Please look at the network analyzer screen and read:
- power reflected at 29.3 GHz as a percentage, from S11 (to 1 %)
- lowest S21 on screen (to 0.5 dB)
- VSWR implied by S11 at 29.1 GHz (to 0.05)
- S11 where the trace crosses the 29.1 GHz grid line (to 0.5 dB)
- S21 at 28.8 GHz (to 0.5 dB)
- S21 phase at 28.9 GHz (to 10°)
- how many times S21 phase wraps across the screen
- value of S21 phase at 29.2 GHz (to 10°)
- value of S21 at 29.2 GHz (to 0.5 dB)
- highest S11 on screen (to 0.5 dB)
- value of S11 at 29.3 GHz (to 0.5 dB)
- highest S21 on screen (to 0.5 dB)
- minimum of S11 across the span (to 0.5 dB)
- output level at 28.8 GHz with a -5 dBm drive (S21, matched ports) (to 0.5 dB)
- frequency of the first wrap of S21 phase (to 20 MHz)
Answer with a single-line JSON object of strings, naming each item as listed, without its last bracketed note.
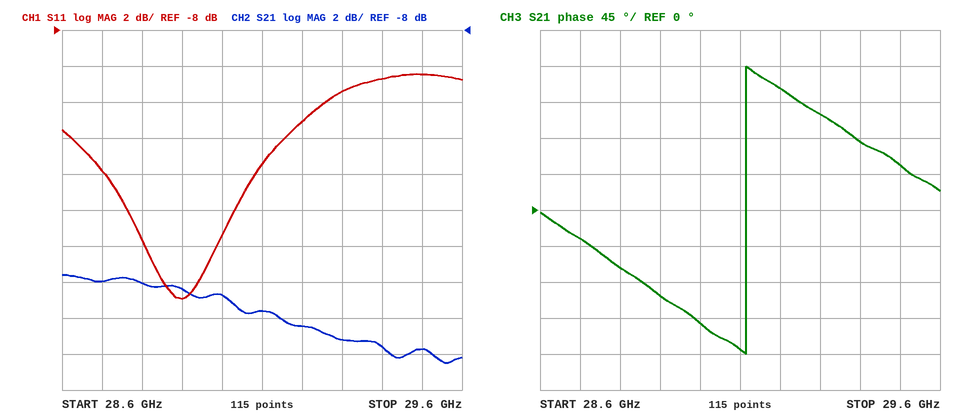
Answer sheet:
{"power reflected at 29.3 GHz as a percentage, from S11": "7 %", "lowest S21 on screen": "-26.5 dB", "VSWR implied by S11 at 29.1 GHz": "1.40", "S11 where the trace crosses the 29.1 GHz grid line": "-15.5 dB", "S21 at 28.8 GHz": "-22.0 dB", "S21 phase at 28.9 GHz": "-110°", "how many times S21 phase wraps across the screen": "1", "value of S21 phase at 29.2 GHz": "150°", "value of S21 at 29.2 GHz": "-24.5 dB", "highest S11 on screen": "-10.5 dB", "value of S11 at 29.3 GHz": "-11.5 dB", "highest S21 on screen": "-21.5 dB", "minimum of S11 across the span": "-23.0 dB", "output level at 28.8 GHz with a -5 dBm drive (S21, matched ports)": "-27.0 dBm", "frequency of the first wrap of S21 phase": "29.12 GHz"}
